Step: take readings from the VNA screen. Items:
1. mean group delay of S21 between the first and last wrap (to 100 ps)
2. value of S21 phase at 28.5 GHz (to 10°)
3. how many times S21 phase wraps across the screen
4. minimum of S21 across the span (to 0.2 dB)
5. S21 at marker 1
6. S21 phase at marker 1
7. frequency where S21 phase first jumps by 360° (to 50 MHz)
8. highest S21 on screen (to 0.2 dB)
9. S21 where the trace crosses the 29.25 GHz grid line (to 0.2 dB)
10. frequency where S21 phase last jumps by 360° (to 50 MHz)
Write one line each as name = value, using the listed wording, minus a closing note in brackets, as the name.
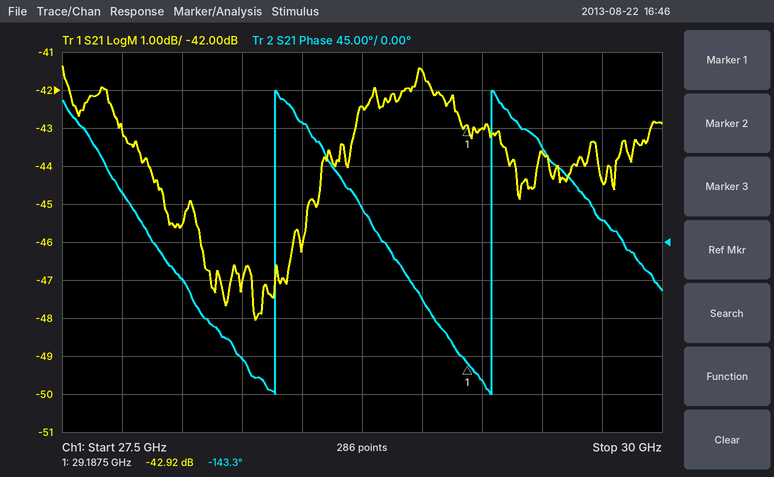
mean group delay of S21 between the first and last wrap = 1.1 ns
value of S21 phase at 28.5 GHz = 140°
how many times S21 phase wraps across the screen = 2
minimum of S21 across the span = -48.0 dB
S21 at marker 1 = -42.92 dB
S21 phase at marker 1 = -143.3°
frequency where S21 phase first jumps by 360° = 28.40 GHz
highest S21 on screen = -41.4 dB
S21 where the trace crosses the 29.25 GHz grid line = -43.0 dB
frequency where S21 phase last jumps by 360° = 29.30 GHz
